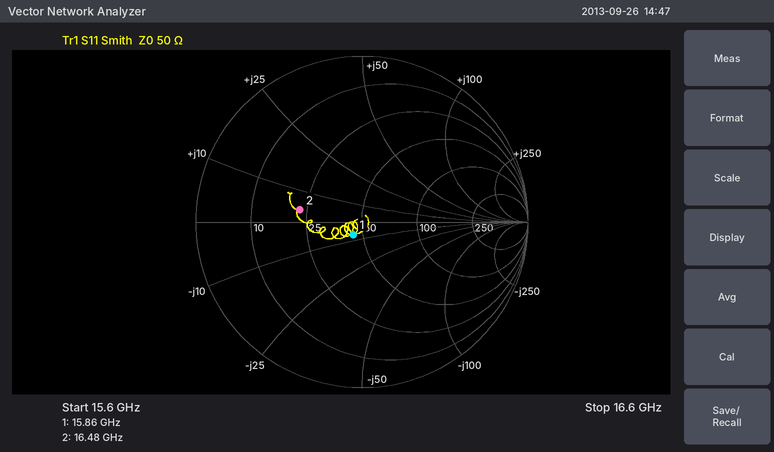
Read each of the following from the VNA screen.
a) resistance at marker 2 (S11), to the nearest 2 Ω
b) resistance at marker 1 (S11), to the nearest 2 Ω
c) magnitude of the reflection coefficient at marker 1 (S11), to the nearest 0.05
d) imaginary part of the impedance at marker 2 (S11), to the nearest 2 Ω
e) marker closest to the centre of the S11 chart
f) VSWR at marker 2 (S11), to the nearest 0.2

22 Ω
44 Ω
0.10
+4 Ω
marker 1
2.2
